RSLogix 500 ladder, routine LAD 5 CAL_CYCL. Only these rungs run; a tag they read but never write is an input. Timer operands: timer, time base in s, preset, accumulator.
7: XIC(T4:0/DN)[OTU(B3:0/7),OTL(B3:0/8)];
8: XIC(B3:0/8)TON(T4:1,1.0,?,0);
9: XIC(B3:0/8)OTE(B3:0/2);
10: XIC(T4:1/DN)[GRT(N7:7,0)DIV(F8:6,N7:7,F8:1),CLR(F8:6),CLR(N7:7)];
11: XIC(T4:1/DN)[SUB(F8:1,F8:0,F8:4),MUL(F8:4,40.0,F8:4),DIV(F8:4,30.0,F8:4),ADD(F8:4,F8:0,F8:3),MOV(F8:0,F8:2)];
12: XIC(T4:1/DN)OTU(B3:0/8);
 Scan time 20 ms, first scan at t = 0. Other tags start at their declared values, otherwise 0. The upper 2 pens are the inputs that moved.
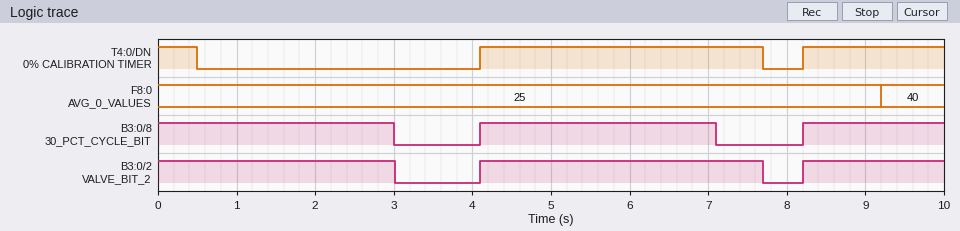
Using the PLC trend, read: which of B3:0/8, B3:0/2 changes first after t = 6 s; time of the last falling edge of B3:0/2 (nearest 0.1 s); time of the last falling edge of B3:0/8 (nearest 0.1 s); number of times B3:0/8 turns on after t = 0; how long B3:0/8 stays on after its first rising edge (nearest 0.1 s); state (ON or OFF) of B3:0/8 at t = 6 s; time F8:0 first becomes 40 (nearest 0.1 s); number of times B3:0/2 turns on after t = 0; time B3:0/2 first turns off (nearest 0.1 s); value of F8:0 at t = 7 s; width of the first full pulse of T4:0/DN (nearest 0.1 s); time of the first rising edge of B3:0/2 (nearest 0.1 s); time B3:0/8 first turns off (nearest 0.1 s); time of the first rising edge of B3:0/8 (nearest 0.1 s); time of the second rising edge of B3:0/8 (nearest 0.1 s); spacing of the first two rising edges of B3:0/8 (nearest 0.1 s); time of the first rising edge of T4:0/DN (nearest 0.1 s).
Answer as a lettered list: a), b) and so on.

a) B3:0/8
b) 7.7 s
c) 7.1 s
d) 2
e) 3.0 s
f) ON
g) 9.2 s
h) 2
i) 3.0 s
j) 25
k) 3.6 s
l) 4.1 s
m) 3.0 s
n) 4.1 s
o) 8.2 s
p) 4.1 s
q) 4.1 s
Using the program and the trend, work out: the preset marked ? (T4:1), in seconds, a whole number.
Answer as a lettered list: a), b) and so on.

a) 3 s
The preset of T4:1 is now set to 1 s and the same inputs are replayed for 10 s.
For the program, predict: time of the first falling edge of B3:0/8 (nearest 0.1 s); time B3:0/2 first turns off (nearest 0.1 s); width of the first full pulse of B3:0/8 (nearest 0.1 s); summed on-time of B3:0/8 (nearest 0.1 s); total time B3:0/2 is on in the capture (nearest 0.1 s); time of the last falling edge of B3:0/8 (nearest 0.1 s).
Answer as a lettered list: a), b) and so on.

a) 1.0 s
b) 1.0 s
c) 1.0 s
d) 3.0 s
e) 6.4 s
f) 9.2 s
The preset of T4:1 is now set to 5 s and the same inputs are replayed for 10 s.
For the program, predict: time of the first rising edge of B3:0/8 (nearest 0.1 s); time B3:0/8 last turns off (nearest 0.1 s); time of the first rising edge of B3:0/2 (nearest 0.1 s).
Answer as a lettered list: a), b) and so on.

a) 8.2 s
b) 5.0 s
c) 8.2 s
